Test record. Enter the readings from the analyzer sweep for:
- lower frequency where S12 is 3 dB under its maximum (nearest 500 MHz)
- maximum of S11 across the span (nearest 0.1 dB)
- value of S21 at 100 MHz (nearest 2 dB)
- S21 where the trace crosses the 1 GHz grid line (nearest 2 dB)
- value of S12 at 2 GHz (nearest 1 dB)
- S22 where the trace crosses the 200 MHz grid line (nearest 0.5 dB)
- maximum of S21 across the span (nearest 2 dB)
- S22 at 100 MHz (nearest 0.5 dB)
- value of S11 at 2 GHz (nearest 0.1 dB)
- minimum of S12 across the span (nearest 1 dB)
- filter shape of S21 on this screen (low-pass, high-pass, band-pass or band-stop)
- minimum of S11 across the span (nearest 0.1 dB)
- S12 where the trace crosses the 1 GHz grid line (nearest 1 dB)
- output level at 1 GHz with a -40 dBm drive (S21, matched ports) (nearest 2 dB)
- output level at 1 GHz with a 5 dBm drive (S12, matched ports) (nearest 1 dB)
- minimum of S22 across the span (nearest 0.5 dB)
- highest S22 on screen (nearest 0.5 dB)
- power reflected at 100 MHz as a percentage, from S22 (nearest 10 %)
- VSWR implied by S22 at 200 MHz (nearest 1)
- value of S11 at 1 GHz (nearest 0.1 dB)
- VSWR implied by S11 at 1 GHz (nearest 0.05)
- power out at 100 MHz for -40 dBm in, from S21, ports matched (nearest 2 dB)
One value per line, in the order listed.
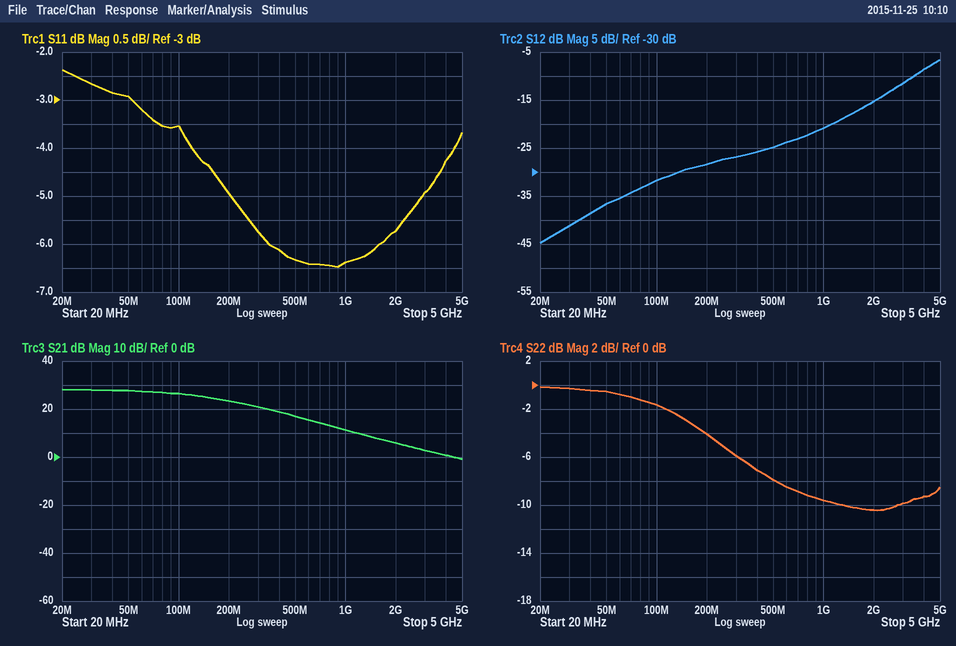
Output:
3.5 GHz
-2.4 dB
26 dB
12 dB
-15 dB
-4.0 dB
28 dB
-1.5 dB
-5.7 dB
-45 dB
low-pass
-6.5 dB
-21 dB
-28 dBm
-16 dBm
-10.5 dB
0.0 dB
70 %
4
-6.4 dB
2.85
-14 dBm
